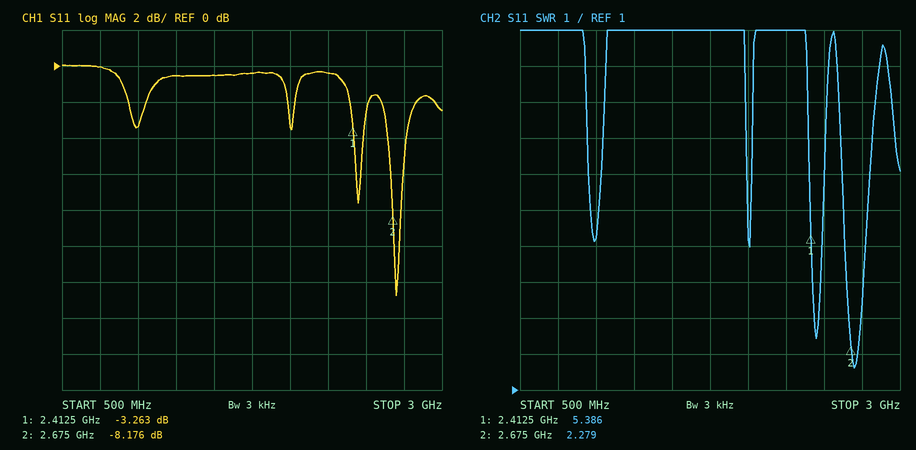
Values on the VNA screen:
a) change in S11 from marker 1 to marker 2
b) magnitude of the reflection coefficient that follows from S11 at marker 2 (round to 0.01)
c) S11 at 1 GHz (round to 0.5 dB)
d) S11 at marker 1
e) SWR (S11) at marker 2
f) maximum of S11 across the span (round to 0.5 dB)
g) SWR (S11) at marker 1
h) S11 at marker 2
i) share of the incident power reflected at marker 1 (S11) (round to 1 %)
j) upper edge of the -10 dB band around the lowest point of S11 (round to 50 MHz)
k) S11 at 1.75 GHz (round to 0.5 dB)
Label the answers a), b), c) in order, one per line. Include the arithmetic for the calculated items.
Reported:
a) -8.176 − (-3.263) = -4.913 dB
b) 10^(-8.176/20) ≈ 0.39
c) -3.5 dB
d) -3.263 dB
e) 2.279
f) 0.0 dB
g) 5.386
h) -8.176 dB
i) 10^(-3.263/10) ≈ 47 %
j) 2.70 GHz
k) -0.5 dB
